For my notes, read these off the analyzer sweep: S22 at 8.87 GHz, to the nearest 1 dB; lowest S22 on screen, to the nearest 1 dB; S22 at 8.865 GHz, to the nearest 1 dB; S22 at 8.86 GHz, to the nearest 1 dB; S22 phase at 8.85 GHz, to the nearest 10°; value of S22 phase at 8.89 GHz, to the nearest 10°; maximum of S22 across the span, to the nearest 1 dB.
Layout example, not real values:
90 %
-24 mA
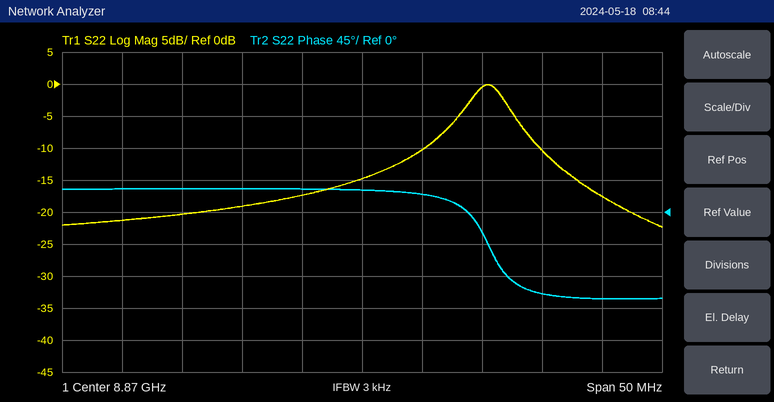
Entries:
-15 dB
-22 dB
-17 dB
-19 dB
30°
-120°
0 dB
